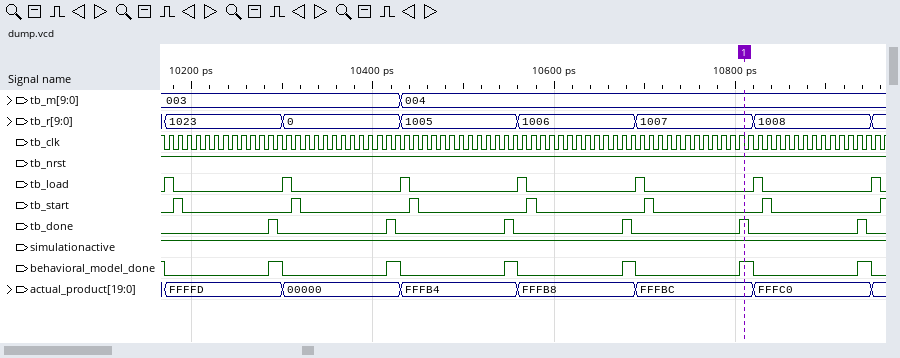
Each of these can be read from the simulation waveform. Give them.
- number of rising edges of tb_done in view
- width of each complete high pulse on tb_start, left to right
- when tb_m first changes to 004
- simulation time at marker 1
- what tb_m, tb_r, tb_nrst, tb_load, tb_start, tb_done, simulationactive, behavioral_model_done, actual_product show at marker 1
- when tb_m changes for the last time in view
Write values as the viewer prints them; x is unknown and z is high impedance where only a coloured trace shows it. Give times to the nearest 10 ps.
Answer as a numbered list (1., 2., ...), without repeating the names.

1. 6
2. 10 ps, 10 ps, 10 ps, 10 ps, 10 ps, 10 ps
3. 10430 ps
4. 10810 ps
5. tb_m=004, tb_r=1007, tb_nrst=1, tb_load=0, tb_start=0, tb_done=1, simulationactive=1, behavioral_model_done=1, actual_product=FFFBC
6. 10430 ps
